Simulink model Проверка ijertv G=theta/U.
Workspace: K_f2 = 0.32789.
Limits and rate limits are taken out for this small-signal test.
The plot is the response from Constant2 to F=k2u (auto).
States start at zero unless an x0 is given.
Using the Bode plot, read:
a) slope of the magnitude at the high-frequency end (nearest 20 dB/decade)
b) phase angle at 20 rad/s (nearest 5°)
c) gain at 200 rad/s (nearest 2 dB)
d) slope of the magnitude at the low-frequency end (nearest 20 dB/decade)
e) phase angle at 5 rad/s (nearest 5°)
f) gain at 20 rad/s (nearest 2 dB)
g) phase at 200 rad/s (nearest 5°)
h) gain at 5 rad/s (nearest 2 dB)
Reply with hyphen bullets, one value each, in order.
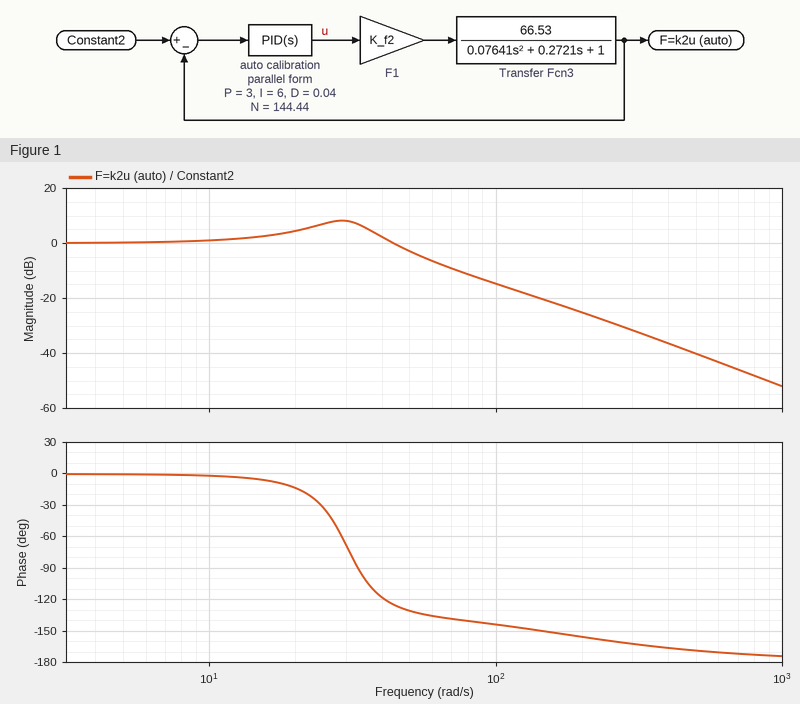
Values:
- -40 dB/decade
- -15°
- -26 dB
- 0 dB/decade
- 0°
- 4 dB
- -155°
- 0 dB
